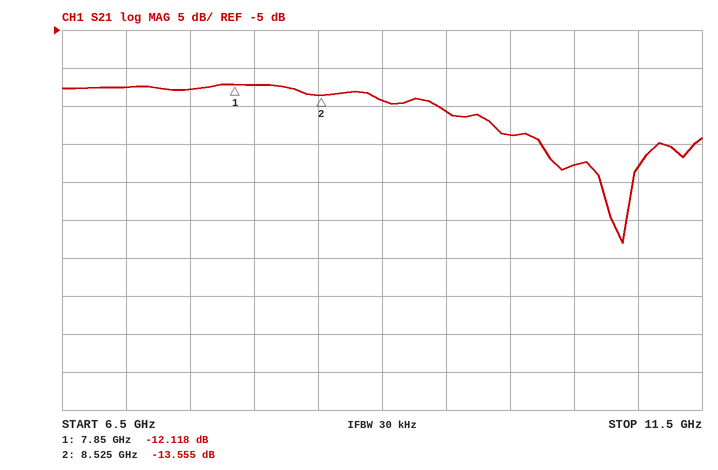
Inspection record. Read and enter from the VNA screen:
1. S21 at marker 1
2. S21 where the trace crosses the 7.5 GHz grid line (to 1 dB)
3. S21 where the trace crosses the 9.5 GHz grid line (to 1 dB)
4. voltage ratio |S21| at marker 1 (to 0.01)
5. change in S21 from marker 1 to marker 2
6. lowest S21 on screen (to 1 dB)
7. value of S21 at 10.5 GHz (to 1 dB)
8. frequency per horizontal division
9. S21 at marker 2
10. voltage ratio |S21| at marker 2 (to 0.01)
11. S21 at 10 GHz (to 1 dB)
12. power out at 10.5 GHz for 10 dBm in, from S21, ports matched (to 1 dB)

-12.118 dB
-13 dB
-16 dB
0.25
-1.437 dB
-33 dB
-23 dB
500 MHz
-13.555 dB
0.21
-19 dB
-13 dBm
